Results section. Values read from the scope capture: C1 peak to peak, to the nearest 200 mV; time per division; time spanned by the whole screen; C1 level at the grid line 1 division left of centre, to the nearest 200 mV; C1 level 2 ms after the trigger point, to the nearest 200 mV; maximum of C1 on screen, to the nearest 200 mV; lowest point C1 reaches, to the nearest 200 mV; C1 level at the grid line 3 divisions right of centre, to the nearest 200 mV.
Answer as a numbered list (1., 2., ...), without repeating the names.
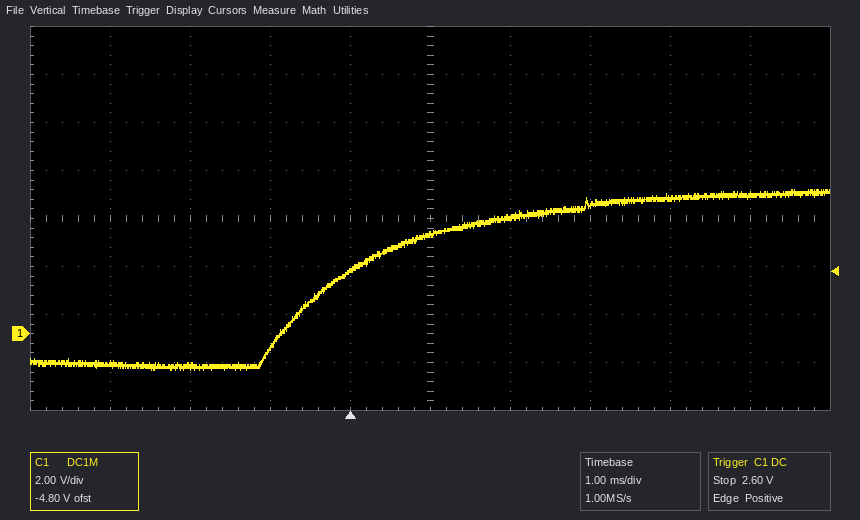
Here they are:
1. 7.6 V
2. 1 ms
3. 10 ms
4. 2.6 V
5. 4.8 V
6. 6.0 V
7. -1.6 V
8. 5.6 V
